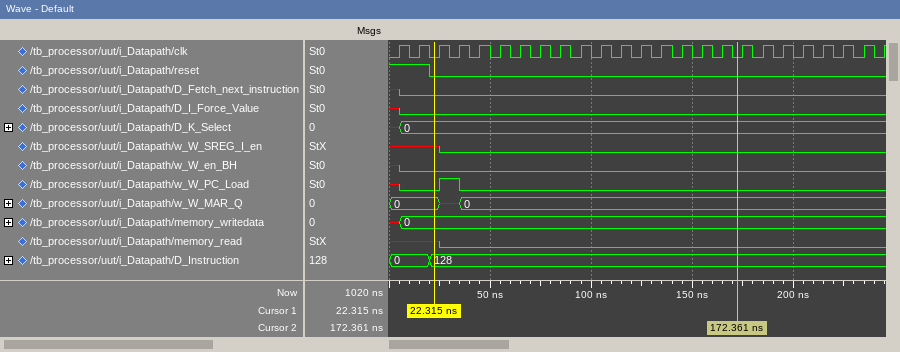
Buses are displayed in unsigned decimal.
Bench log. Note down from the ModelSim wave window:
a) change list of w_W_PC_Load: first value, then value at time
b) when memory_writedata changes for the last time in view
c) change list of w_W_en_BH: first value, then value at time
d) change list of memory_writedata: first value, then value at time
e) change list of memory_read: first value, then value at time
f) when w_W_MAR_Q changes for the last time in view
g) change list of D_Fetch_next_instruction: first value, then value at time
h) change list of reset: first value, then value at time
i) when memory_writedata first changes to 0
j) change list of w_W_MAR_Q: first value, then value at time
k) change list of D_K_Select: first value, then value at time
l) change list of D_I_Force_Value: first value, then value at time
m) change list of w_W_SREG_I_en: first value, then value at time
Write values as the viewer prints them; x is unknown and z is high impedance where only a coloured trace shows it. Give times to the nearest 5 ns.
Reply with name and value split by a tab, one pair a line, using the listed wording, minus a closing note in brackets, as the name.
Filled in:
change list of w_W_PC_Load: first value, then value at time	x, 0 at 5 ns, 1 at 25 ns, 0 at 35 ns
when memory_writedata changes for the last time in view	5 ns
change list of w_W_en_BH: first value, then value at time	x, 0 at 5 ns
change list of memory_writedata: first value, then value at time	x, 0 at 5 ns
change list of memory_read: first value, then value at time	x, 0 at 25 ns
when w_W_MAR_Q changes for the last time in view	35 ns
change list of D_Fetch_next_instruction: first value, then value at time	x, 0 at 5 ns
change list of reset: first value, then value at time	1, 0 at 20 ns
when memory_writedata first changes to 0	5 ns
change list of w_W_MAR_Q: first value, then value at time	0, x at 25 ns, 0 at 35 ns
change list of D_K_Select: first value, then value at time	x, 0 at 5 ns
change list of D_I_Force_Value: first value, then value at time	x, 0 at 5 ns
change list of w_W_SREG_I_en: first value, then value at time	x, 0 at 25 ns
